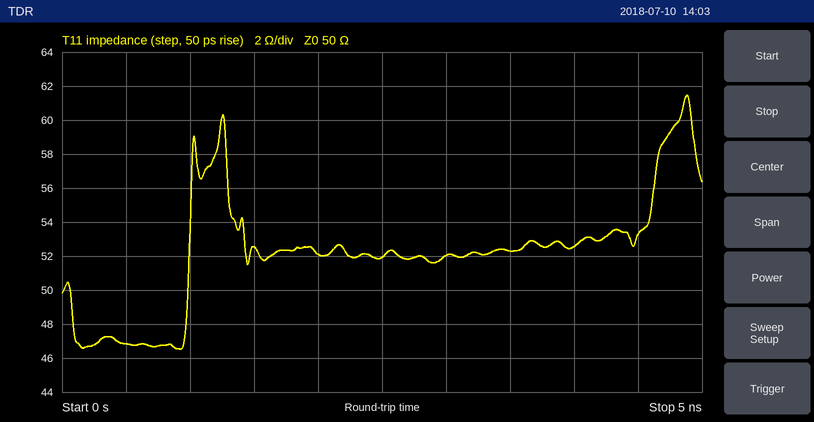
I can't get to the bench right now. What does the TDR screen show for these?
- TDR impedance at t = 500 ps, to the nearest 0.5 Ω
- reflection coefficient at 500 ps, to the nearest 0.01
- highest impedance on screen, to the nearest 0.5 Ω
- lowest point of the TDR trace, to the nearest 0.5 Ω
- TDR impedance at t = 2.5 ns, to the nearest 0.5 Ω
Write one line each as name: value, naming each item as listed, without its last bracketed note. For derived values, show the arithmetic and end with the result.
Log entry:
TDR impedance at t = 500 ps, to the nearest 0.5 Ω: 47.0 Ω
reflection coefficient at 500 ps, to the nearest 0.01: (47 − 50)/(47 + 50) ≈ -0.03
highest impedance on screen, to the nearest 0.5 Ω: 61.5 Ω
lowest point of the TDR trace, to the nearest 0.5 Ω: 46.5 Ω
TDR impedance at t = 2.5 ns, to the nearest 0.5 Ω: 52.0 Ω
